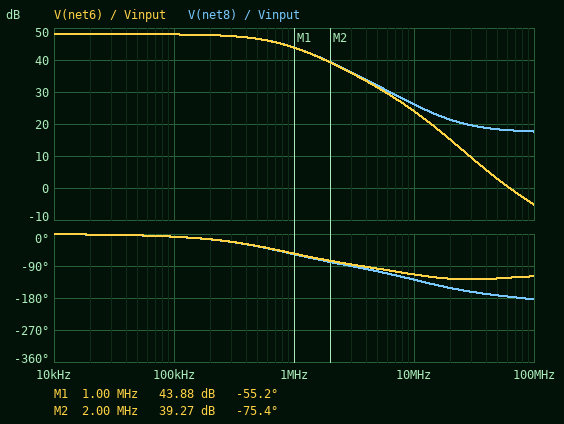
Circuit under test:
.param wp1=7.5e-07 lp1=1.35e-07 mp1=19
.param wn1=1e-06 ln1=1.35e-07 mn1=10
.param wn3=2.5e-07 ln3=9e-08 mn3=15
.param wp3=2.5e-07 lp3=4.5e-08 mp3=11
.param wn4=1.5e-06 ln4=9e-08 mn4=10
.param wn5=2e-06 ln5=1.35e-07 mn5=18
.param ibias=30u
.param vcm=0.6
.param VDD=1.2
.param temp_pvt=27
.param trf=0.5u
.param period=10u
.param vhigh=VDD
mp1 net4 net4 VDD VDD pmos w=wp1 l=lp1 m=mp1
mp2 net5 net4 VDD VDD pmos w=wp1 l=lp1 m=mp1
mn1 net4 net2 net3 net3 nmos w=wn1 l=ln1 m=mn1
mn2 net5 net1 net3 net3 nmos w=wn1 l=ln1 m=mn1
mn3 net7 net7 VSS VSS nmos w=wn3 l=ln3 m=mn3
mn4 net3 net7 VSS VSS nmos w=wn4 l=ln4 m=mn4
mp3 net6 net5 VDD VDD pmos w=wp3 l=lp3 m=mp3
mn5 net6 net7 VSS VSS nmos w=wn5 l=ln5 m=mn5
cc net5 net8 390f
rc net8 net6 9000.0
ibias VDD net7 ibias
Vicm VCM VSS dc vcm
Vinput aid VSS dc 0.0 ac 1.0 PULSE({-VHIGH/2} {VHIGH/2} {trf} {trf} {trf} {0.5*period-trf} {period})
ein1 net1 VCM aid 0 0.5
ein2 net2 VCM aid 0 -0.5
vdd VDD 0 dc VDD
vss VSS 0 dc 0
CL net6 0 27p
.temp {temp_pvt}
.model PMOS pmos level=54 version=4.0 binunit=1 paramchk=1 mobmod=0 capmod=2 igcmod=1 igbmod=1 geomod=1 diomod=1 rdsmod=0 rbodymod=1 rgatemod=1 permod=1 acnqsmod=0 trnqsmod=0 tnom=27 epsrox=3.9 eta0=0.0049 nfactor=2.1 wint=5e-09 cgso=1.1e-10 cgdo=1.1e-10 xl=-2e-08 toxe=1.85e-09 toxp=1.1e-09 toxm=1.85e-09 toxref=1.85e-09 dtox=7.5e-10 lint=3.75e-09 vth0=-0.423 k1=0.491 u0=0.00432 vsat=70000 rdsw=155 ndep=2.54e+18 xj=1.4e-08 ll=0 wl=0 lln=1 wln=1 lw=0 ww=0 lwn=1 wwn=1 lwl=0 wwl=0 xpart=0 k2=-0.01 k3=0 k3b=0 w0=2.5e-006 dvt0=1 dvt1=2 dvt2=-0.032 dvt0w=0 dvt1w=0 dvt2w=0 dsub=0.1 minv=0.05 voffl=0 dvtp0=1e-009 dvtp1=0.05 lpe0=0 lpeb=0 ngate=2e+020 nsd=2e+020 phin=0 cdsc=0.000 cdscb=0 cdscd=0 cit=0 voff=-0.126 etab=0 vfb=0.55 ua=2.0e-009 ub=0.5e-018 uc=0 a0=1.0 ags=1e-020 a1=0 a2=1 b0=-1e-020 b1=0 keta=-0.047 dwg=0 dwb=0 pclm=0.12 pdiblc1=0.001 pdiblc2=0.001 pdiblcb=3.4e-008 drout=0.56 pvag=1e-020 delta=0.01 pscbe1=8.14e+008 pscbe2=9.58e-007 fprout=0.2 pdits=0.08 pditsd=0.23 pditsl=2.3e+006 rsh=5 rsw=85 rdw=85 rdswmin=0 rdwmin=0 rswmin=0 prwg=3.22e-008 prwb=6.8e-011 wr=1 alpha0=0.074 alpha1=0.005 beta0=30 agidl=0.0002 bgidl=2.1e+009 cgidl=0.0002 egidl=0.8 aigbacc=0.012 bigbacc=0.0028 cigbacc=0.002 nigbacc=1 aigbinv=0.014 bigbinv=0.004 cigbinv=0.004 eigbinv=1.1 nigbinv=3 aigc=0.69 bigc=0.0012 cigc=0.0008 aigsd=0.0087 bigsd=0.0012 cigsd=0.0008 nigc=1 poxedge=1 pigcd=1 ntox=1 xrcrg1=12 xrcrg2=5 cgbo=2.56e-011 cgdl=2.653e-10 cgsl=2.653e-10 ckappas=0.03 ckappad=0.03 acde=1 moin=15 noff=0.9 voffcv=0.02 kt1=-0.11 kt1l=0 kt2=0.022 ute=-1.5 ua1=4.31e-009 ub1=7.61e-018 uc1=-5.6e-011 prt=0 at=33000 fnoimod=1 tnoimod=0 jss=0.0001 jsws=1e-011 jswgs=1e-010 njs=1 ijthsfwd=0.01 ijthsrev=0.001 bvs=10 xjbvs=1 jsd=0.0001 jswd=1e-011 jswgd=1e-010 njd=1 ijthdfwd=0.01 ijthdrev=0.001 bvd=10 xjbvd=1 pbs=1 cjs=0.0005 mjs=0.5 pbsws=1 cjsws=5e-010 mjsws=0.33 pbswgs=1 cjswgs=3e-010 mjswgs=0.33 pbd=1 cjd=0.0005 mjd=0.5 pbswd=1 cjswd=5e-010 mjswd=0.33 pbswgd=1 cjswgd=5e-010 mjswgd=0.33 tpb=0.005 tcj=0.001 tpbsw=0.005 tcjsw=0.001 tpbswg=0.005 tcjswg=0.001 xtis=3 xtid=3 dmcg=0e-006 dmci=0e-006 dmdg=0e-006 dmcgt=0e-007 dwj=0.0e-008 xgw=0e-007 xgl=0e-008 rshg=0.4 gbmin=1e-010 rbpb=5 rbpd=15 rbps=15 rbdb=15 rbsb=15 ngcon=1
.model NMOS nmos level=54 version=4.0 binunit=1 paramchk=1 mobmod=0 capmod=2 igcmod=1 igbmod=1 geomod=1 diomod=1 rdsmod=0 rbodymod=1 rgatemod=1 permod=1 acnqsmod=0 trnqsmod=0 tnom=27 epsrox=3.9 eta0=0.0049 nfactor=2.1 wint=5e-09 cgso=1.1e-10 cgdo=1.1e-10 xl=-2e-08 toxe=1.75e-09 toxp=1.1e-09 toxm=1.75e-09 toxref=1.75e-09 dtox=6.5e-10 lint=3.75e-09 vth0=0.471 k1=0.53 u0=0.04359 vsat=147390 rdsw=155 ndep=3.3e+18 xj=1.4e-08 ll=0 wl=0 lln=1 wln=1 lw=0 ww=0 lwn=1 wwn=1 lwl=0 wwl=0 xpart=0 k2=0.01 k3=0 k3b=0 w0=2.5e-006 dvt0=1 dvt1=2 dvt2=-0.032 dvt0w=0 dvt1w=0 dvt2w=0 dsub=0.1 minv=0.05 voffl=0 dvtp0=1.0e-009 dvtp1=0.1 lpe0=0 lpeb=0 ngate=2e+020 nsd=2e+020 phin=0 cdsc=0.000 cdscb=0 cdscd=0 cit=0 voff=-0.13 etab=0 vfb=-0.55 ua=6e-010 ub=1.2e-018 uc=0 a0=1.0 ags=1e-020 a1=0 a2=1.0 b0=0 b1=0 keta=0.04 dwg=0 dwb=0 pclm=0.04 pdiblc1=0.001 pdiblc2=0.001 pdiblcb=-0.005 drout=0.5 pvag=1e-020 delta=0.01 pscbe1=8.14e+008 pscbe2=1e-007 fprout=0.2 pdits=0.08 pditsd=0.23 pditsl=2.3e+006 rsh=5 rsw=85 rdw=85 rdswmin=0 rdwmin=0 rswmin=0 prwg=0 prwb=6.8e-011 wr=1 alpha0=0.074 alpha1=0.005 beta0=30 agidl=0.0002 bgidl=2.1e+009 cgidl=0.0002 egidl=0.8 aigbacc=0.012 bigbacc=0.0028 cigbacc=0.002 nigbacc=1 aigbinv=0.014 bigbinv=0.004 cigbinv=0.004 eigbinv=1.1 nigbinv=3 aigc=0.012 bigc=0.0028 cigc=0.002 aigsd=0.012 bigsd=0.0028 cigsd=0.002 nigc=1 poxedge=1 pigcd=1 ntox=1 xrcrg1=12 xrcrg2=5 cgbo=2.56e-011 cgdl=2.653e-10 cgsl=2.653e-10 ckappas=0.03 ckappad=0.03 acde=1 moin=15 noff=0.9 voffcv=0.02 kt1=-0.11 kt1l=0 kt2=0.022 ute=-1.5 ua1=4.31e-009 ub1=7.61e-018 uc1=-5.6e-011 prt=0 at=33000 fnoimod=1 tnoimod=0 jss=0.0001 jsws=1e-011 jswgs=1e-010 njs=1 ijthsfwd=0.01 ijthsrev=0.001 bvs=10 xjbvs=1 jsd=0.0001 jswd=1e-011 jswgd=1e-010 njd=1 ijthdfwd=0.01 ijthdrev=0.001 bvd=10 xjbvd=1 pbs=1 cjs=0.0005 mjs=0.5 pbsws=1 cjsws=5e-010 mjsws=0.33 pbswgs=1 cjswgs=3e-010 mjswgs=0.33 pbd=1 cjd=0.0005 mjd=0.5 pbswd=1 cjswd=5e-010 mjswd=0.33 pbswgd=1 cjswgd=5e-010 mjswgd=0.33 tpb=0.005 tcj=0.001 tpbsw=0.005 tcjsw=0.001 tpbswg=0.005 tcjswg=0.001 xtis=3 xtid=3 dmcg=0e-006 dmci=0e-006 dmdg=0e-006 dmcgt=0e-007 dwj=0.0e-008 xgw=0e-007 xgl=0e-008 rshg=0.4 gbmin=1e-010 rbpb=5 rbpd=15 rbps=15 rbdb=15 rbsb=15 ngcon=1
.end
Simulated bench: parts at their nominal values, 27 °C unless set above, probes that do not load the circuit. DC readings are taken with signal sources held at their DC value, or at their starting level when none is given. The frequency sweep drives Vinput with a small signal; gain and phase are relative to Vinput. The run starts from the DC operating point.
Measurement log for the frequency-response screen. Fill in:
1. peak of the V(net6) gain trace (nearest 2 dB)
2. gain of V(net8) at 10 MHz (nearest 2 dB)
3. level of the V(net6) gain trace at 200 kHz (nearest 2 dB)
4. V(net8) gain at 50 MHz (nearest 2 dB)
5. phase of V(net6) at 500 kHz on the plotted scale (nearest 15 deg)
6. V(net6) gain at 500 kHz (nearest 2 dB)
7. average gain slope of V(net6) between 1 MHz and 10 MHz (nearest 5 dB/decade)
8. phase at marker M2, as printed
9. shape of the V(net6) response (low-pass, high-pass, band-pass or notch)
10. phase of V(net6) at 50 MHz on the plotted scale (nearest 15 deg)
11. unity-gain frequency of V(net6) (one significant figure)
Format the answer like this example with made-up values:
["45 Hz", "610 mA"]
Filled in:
["48 dB", "26 dB", "48 dB", "18 dB", "-30 deg", "46 dB", "-20 dB/decade", "-75.4 deg", "low-pass", "-120 deg", "60 MHz"]
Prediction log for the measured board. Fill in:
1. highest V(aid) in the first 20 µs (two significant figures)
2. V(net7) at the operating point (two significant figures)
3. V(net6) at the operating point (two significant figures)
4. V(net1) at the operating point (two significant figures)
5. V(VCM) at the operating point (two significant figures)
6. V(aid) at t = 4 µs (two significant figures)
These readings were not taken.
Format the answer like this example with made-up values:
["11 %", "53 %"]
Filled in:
["600 mV", "440 mV", "730 mV", "600 mV", "600 mV", "600 mV"]
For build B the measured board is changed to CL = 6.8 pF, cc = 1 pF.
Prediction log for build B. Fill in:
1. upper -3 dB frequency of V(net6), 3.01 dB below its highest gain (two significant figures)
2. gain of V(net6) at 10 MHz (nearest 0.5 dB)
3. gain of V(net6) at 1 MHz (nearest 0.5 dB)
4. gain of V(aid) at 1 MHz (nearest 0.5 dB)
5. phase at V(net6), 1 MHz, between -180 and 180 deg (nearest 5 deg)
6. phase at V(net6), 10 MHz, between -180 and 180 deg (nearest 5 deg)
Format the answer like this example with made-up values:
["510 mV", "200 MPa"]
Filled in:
["450 kHz", "22.0 dB", "40.5 dB", "0 dB", "-65 deg", "-75 deg"]
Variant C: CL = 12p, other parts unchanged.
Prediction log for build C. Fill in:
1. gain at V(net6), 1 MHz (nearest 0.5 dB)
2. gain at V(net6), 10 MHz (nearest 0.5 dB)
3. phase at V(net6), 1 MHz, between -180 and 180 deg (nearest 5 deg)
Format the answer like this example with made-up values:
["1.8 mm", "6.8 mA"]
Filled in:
["45.0 dB", "27.5 dB", "-45 deg"]
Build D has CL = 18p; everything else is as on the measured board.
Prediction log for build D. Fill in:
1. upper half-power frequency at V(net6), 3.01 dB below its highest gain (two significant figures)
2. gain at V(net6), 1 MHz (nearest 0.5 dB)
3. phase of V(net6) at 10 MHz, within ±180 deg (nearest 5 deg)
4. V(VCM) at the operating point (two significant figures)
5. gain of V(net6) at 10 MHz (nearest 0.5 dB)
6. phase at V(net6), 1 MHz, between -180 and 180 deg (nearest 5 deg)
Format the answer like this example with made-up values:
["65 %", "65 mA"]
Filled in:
["900 kHz", "44.5 dB", "-105 deg", "600 mV", "26.0 dB", "-50 deg"]
